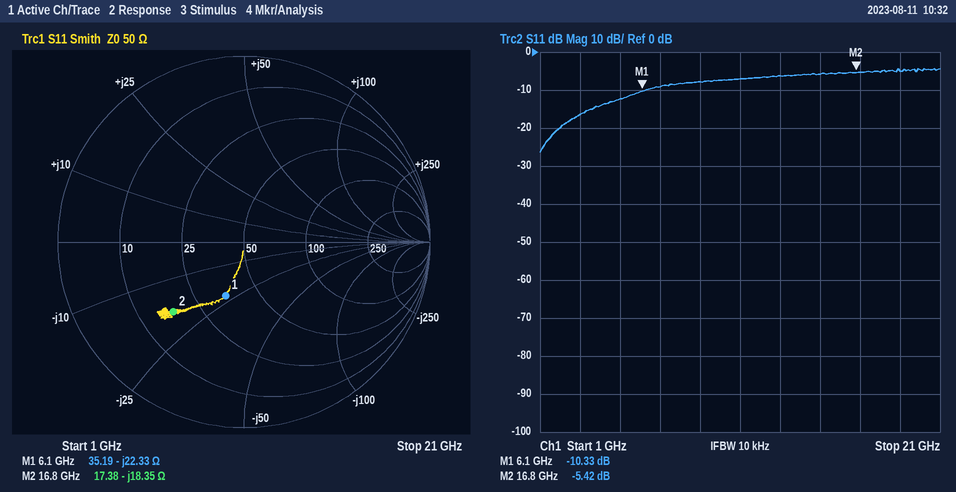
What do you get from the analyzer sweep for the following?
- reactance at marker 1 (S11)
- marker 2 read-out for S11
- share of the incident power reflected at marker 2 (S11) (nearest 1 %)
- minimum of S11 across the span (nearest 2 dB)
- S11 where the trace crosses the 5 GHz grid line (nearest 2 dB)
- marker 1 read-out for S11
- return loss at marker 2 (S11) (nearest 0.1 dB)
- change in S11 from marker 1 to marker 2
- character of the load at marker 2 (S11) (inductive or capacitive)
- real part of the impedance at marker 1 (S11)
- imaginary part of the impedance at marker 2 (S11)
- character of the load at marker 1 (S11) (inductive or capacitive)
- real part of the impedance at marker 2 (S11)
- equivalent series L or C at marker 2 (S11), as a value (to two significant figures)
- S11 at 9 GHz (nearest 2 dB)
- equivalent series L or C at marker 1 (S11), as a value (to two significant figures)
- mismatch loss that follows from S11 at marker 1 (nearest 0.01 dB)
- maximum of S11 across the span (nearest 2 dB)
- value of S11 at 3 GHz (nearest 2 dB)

-22.33 Ω
-5.42 dB
29 %
-26 dB
-12 dB
-10.33 dB
5.4 dB
4.91 dB
capacitive
35.19 Ω
-18.35 Ω
capacitive
17.38 Ω
520 fF
-8 dB
1.2 pF
0.42 dB
-4 dB
-16 dB
